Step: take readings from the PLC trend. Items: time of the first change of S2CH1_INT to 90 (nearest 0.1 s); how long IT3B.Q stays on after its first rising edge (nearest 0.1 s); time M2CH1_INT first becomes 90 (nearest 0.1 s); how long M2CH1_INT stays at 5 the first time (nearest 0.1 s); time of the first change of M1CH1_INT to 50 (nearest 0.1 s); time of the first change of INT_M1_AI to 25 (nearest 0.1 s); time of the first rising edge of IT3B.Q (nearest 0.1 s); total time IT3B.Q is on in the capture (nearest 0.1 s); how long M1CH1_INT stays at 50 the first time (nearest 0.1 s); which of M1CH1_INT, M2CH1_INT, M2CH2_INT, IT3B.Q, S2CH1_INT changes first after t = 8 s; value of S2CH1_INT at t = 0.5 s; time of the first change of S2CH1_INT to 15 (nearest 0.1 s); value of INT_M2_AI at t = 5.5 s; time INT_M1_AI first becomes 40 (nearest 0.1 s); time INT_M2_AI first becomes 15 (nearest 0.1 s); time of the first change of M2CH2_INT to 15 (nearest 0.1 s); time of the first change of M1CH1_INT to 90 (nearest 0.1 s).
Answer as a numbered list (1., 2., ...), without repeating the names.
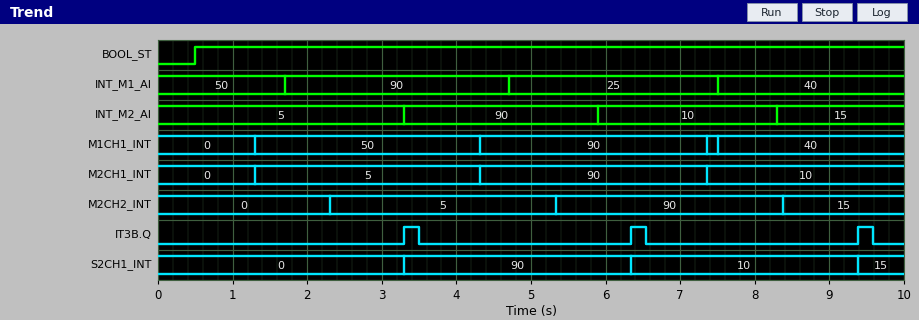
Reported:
1. 3.3 s
2. 0.2 s
3. 4.3 s
4. 3.0 s
5. 1.3 s
6. 4.7 s
7. 3.3 s
8. 0.6 s
9. 3.0 s
10. M2CH2_INT
11. 0
12. 9.4 s
13. 90
14. 7.5 s
15. 8.3 s
16. 8.4 s
17. 4.3 s
